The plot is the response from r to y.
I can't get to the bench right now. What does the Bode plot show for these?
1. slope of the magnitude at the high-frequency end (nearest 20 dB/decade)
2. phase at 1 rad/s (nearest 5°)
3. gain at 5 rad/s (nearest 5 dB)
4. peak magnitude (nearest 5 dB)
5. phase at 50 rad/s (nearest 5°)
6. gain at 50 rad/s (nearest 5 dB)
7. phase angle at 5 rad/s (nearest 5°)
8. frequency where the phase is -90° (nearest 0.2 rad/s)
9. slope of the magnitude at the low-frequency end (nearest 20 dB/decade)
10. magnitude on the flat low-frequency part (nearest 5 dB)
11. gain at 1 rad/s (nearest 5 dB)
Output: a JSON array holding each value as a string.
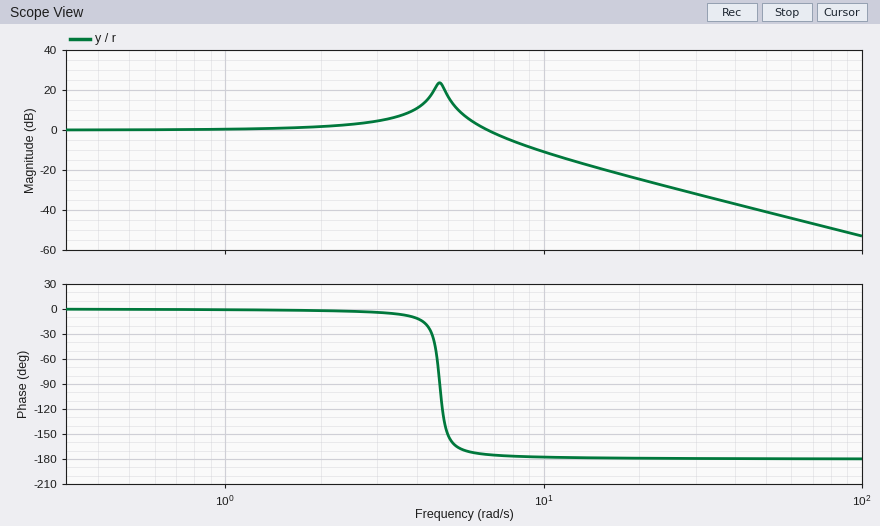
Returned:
["-40 dB/decade", "0°", "15 dB", "25 dB", "-180°", "-40 dB", "-150°", "4.8 rad/s", "0 dB/decade", "0 dB", "0 dB"]
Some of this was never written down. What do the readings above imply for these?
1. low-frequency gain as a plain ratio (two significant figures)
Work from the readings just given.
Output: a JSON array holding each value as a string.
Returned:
["1.0"]
